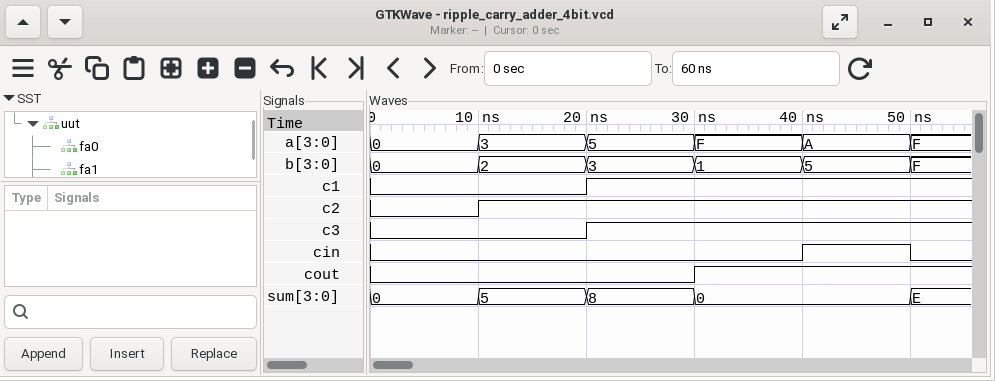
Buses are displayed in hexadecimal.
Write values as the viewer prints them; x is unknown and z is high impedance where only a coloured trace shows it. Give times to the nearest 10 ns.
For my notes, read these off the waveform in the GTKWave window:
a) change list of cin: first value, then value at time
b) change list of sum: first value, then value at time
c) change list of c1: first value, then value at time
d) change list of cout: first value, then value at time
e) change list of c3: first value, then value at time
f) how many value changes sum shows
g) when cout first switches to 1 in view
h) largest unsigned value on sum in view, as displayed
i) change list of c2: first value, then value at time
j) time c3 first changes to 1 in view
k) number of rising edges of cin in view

0, 1 at 40 ns, 0 at 50 ns
0, 5 at 10 ns, 8 at 20 ns, 0 at 30 ns, E at 50 ns
0, 1 at 20 ns
0, 1 at 30 ns
0, 1 at 20 ns
4
30 ns
E
0, 1 at 10 ns
20 ns
1
